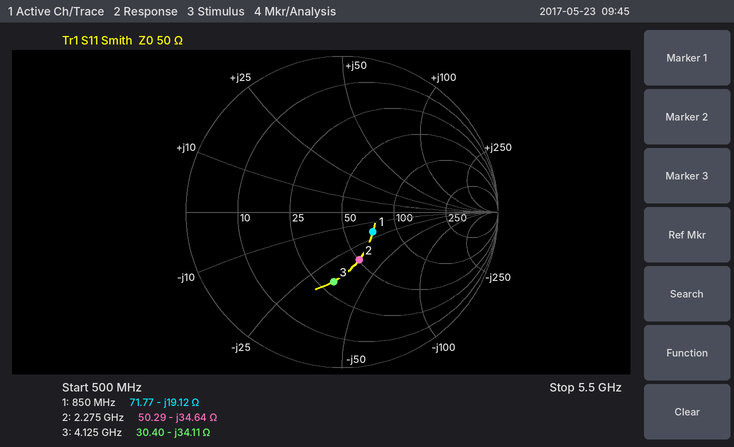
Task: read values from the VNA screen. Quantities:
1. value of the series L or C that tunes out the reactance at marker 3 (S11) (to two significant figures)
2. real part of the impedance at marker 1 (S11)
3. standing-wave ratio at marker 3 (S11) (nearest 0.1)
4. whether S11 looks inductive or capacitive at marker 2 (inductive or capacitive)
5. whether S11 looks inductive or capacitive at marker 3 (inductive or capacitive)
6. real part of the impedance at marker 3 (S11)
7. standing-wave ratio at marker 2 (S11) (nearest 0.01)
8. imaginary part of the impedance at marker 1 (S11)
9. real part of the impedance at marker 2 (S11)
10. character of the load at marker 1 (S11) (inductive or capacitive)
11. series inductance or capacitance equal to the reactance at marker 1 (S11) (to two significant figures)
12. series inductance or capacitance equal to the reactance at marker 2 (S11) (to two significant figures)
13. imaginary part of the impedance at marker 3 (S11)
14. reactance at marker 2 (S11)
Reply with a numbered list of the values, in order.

1. 1.3 nH
2. 71.77 Ω
3. 2.6
4. capacitive
5. capacitive
6. 30.40 Ω
7. 1.97
8. -19.12 Ω
9. 50.29 Ω
10. capacitive
11. 9.8 pF
12. 2.0 pF
13. -34.11 Ω
14. -34.64 Ω
